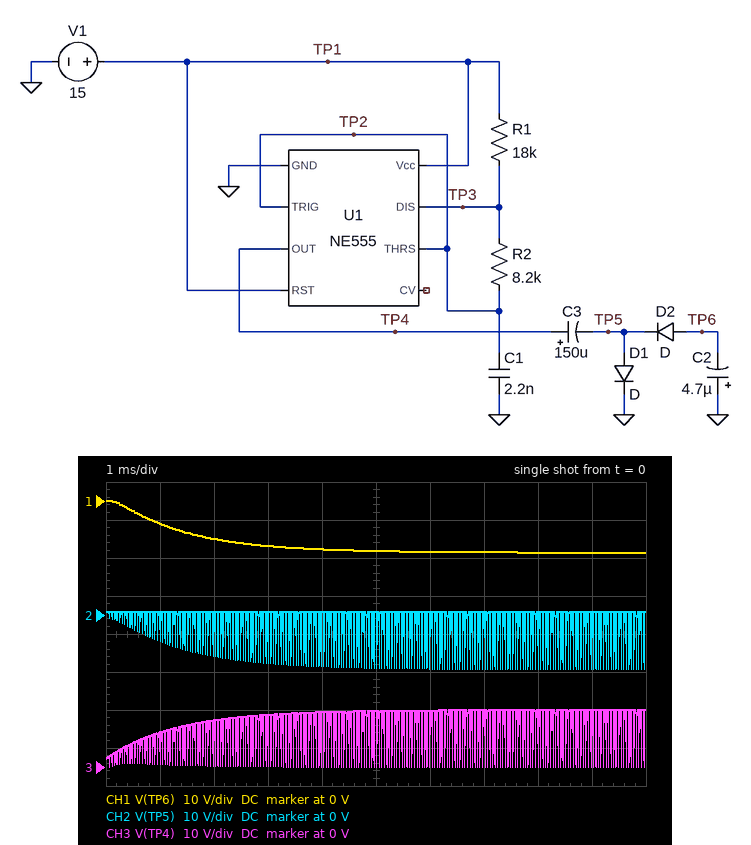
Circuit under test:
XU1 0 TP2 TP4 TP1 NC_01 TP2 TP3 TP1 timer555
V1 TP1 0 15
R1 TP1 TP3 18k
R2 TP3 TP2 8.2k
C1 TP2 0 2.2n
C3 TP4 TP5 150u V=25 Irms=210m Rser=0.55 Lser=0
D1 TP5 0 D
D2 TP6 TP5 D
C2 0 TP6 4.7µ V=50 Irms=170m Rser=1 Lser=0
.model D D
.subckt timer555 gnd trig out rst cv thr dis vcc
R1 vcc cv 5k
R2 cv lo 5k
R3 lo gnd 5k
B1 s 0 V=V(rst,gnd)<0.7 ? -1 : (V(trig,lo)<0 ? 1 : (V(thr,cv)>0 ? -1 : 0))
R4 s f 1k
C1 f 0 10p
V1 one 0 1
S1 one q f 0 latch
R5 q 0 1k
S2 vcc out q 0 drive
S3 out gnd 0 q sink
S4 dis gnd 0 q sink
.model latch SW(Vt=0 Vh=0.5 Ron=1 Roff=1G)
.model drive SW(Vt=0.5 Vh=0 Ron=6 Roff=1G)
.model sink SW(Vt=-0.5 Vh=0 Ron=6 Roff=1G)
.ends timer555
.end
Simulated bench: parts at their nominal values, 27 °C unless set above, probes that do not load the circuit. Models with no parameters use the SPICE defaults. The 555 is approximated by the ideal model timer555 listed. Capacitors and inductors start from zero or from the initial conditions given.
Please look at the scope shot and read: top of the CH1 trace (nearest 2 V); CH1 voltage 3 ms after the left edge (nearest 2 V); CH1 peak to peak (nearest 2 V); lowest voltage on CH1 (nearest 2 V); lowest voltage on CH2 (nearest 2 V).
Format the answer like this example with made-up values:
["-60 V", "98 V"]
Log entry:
["0 V", "-12 V", "14 V", "-14 V", "-14 V"]
